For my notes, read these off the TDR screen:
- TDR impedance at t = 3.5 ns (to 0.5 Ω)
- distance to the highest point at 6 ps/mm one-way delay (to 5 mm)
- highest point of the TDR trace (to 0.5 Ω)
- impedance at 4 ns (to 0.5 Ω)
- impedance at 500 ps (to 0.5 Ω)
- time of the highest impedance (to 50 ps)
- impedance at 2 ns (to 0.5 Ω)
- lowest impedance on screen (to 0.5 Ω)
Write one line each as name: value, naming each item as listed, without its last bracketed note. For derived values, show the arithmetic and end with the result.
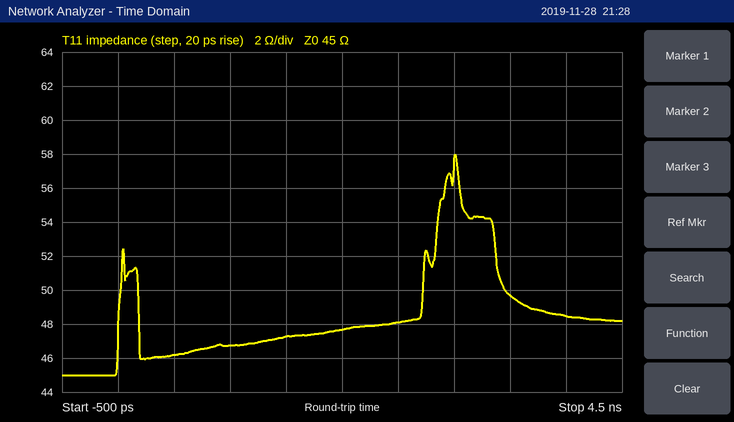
TDR impedance at t = 3.5 ns: 49.5 Ω
distance to the highest point at 6 ps/mm one-way delay: 3.00 ns / 2 / 6 ps/mm ≈ 250 mm
highest point of the TDR trace: 58.0 Ω
impedance at 4 ns: 48.5 Ω
impedance at 500 ps: 46.0 Ω
time of the highest impedance: 3.00 ns
impedance at 2 ns: 47.5 Ω
lowest impedance on screen: 45.0 Ω
